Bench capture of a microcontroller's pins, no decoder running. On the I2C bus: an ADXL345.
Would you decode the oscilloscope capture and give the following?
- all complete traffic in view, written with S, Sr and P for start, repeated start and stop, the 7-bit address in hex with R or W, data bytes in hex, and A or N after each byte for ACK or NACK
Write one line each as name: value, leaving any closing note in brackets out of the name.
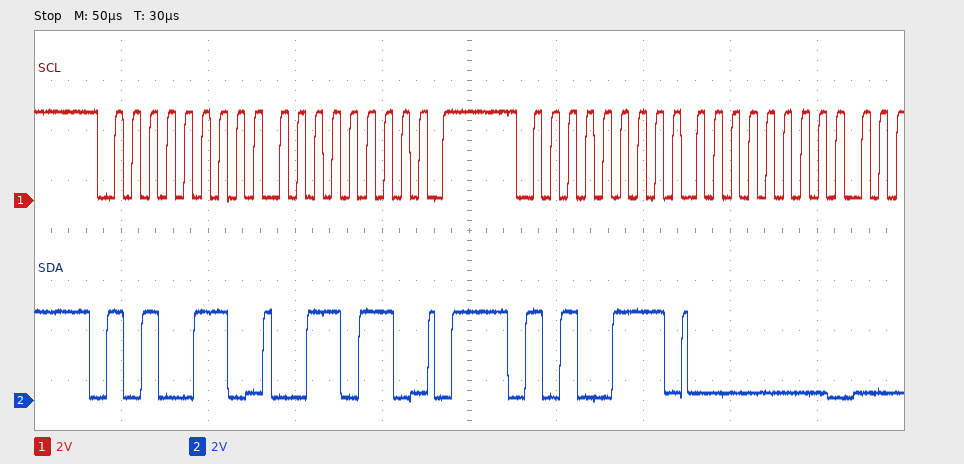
all complete traffic in view, written with S, Sr and P for start, repeated start and stop, the 7-bit address in hex with R or W, data bytes in hex, and A or N after each byte for ACK or NACK: S 53W A 36 A P S 53R A 00 A
